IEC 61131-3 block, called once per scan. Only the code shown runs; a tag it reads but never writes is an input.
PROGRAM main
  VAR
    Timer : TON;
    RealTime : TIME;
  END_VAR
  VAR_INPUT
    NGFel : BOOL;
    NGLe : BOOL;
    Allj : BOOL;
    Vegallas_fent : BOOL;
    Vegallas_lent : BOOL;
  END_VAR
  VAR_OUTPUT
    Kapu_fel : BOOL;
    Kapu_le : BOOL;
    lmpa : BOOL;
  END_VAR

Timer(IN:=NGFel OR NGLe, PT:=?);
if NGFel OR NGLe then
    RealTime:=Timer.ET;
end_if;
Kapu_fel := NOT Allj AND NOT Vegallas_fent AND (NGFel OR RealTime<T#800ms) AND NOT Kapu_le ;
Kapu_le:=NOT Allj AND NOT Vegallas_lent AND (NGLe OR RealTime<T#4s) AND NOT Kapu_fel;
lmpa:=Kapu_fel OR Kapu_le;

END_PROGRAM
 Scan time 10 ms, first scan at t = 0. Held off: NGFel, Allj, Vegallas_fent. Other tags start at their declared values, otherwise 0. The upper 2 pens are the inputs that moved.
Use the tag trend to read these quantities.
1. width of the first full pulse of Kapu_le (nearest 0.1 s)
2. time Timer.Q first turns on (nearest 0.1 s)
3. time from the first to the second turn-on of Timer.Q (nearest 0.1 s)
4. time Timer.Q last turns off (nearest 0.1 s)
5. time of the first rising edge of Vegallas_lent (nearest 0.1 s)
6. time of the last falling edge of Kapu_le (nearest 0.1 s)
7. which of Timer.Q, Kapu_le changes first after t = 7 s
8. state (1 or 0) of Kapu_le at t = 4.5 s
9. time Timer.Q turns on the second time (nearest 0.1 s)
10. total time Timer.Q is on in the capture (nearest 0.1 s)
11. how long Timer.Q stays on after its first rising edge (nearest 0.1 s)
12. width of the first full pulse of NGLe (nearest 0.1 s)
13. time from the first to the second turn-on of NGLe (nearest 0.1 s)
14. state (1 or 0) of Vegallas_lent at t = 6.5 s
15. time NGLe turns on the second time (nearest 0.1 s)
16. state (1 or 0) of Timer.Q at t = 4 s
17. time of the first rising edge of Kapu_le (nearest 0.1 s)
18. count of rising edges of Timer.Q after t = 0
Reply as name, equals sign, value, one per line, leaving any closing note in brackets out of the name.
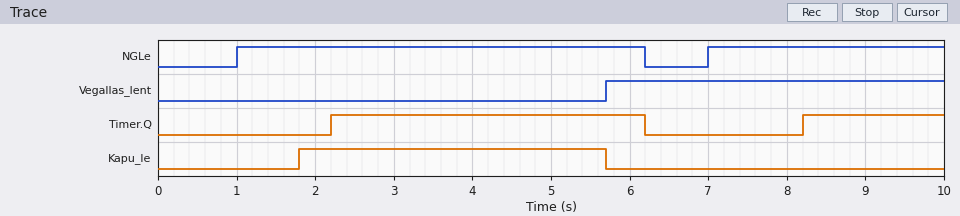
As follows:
width of the first full pulse of Kapu_le = 3.9 s
time Timer.Q first turns on = 2.2 s
time from the first to the second turn-on of Timer.Q = 6.0 s
time Timer.Q last turns off = 6.2 s
time of the first rising edge of Vegallas_lent = 5.7 s
time of the last falling edge of Kapu_le = 5.7 s
which of Timer.Q, Kapu_le changes first after t = 7 s = Timer.Q
state (1 or 0) of Kapu_le at t = 4.5 s = 1
time Timer.Q turns on the second time = 8.2 s
total time Timer.Q is on in the capture = 5.8 s
how long Timer.Q stays on after its first rising edge = 4.0 s
width of the first full pulse of NGLe = 5.2 s
time from the first to the second turn-on of NGLe = 6.0 s
state (1 or 0) of Vegallas_lent at t = 6.5 s = 1
time NGLe turns on the second time = 7.0 s
state (1 or 0) of Timer.Q at t = 4 s = 1
time of the first rising edge of Kapu_le = 1.8 s
count of rising edges of Timer.Q after t = 0 = 2
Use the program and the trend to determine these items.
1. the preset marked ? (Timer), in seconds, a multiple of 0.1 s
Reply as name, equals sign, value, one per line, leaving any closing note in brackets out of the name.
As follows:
the preset marked ? (Timer), in seconds, a multiple of 0.1 s = 1.2 s
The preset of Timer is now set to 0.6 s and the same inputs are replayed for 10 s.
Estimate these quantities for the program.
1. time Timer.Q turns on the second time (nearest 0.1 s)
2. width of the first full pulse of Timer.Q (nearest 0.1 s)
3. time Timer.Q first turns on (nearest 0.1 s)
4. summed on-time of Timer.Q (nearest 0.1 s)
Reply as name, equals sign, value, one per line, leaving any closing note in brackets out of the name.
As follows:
time Timer.Q turns on the second time = 7.6 s
width of the first full pulse of Timer.Q = 4.6 s
time Timer.Q first turns on = 1.6 s
summed on-time of Timer.Q = 7.0 s
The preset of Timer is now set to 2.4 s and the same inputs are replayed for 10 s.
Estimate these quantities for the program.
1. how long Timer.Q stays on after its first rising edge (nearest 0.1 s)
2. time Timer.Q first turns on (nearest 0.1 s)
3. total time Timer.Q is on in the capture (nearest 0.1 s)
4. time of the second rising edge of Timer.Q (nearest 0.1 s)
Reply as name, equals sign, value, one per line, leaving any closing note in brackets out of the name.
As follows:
how long Timer.Q stays on after its first rising edge = 2.8 s
time Timer.Q first turns on = 3.4 s
total time Timer.Q is on in the capture = 3.4 s
time of the second rising edge of Timer.Q = 9.4 s
